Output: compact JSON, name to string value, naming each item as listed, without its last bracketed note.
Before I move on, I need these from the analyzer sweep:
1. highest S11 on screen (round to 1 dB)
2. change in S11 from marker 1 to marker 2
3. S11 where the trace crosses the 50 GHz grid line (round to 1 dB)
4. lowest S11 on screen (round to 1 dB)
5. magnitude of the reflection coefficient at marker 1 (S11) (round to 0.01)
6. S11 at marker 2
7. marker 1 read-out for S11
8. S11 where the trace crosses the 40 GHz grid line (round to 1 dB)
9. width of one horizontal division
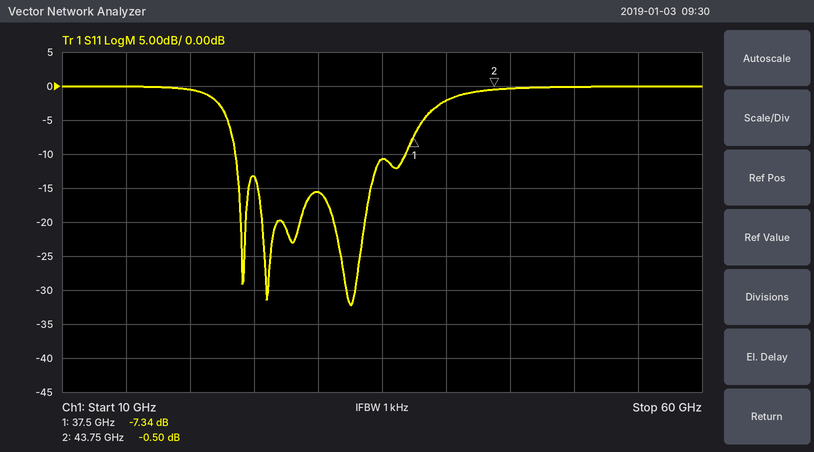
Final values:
{"highest S11 on screen": "0 dB", "change in S11 from marker 1 to marker 2": "6.84 dB", "S11 where the trace crosses the 50 GHz grid line": "0 dB", "lowest S11 on screen": "-32 dB", "magnitude of the reflection coefficient at marker 1 (S11)": "0.43", "S11 at marker 2": "-0.50 dB", "marker 1 read-out for S11": "-7.34 dB", "S11 where the trace crosses the 40 GHz grid line": "-2 dB", "width of one horizontal division": "5 GHz"}
